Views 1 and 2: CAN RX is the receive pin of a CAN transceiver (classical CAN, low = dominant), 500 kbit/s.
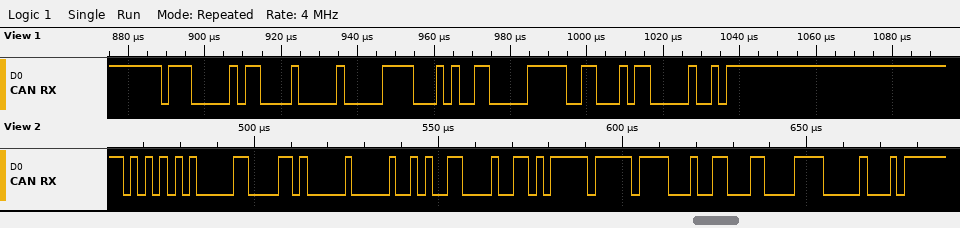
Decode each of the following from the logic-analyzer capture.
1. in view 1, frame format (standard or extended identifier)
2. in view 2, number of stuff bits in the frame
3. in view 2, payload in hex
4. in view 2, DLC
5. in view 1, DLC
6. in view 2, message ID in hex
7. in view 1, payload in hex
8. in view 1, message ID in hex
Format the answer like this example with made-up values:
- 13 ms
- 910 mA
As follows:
- standard
- 6
- 68 00 53 09 AF FF C4 C6
- 8
- 4
- 0x554
- 00 E2 98 3D
- 0x703
